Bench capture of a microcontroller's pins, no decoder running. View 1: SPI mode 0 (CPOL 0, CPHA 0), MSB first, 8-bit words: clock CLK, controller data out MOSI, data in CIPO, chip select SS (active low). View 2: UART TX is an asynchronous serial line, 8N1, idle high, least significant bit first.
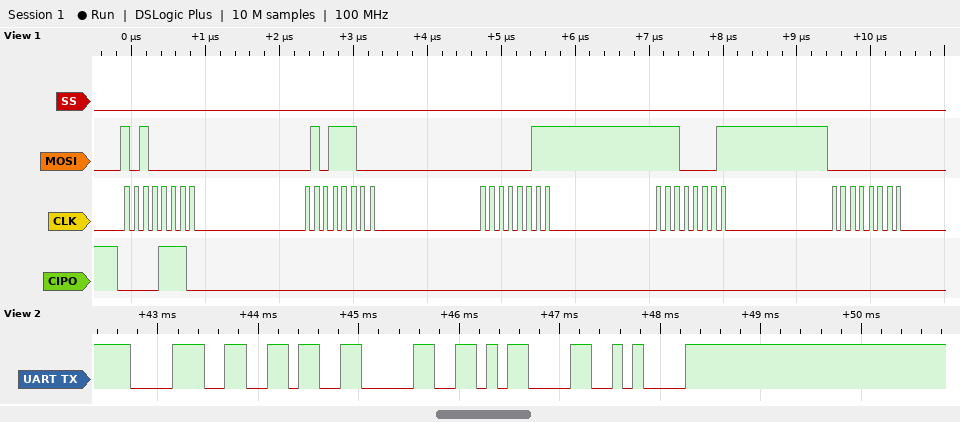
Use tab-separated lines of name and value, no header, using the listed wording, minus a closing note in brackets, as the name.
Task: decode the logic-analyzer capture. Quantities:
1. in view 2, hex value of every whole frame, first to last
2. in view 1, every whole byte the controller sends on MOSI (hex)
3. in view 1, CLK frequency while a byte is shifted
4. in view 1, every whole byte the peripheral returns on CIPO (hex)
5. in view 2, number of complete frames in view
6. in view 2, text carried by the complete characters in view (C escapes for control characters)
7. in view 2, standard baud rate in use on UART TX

in view 2, hex value of every whole frame, first to last	38 36 30 0D 0A
in view 1, every whole byte the controller sends on MOSI	A0 5C 03 E1 00
in view 1, CLK frequency while a byte is shifted	8 MHz
in view 1, every whole byte the peripheral returns on CIPO	0E 00 00 00 00
in view 2, number of complete frames in view	5
in view 2, text carried by the complete characters in view	"860\r\n"
in view 2, standard baud rate in use on UART TX	9600 baud
